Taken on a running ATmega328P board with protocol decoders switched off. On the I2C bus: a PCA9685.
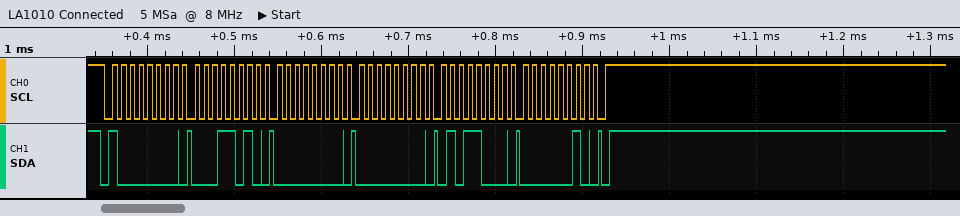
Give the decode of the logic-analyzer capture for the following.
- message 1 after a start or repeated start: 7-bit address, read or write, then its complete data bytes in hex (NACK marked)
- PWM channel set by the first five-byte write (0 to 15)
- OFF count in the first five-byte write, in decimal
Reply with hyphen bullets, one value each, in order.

- 0x40 write: 1A 00 00 58 02
- 5
- 600
